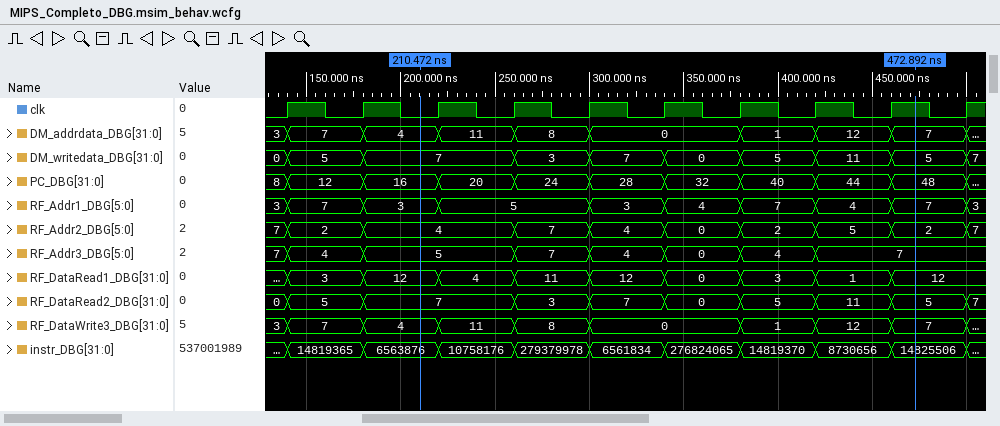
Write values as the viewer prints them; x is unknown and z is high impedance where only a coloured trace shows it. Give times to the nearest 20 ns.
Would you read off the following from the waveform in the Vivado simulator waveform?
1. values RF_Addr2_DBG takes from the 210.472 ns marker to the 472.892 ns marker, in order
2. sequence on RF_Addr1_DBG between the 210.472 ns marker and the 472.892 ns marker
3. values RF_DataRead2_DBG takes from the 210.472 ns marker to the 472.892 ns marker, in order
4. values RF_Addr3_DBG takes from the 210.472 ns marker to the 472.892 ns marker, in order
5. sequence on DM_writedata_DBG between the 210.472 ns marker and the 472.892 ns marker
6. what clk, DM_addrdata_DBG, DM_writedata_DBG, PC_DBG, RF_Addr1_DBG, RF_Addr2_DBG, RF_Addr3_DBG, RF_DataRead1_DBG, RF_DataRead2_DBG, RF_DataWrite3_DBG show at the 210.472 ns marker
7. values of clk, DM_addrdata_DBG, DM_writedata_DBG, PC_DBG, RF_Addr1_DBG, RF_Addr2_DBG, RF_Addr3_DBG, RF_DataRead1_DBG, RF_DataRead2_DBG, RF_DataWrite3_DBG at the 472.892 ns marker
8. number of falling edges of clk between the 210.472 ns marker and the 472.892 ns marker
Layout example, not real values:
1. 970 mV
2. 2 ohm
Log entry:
1. 4, 7, 4, 0, 2, 5, 2
2. 3, 5, 3, 4, 7, 4, 7
3. 7, 3, 7, 0, 5, 11, 5
4. 5, 7, 4, 0, 4, 7
5. 7, 3, 7, 0, 5, 11, 5
6. clk=0, DM_addrdata_DBG=4, DM_writedata_DBG=7, PC_DBG=16, RF_Addr1_DBG=3, RF_Addr2_DBG=4, RF_Addr3_DBG=5, RF_DataRead1_DBG=12, RF_DataRead2_DBG=7, RF_DataWrite3_DBG=4
7. clk=1, DM_addrdata_DBG=7, DM_writedata_DBG=5, PC_DBG=48, RF_Addr1_DBG=7, RF_Addr2_DBG=2, RF_Addr3_DBG=7, RF_DataRead1_DBG=12, RF_DataRead2_DBG=5, RF_DataWrite3_DBG=7
8. 6
